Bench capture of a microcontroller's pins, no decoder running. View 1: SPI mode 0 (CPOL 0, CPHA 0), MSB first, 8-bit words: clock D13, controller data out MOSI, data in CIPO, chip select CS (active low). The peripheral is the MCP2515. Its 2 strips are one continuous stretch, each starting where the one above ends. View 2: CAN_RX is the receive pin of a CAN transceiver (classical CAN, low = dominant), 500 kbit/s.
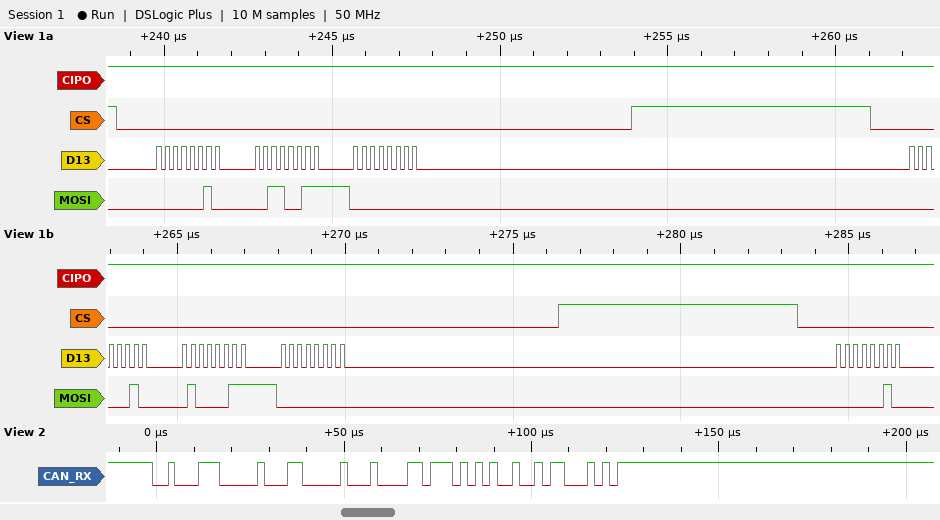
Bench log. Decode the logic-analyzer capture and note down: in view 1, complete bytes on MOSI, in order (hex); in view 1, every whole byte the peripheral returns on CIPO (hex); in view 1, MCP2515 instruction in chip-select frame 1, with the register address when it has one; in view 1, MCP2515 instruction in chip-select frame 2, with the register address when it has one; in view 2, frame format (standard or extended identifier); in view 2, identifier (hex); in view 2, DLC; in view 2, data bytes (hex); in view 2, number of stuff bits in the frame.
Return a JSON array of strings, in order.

["02 33 00 02 43 00 02", "FF FF FF FF FF FF FF", "WRITE 0x33", "WRITE 0x43", "standard", "0x238", "3", "00 86 EA", "2"]
